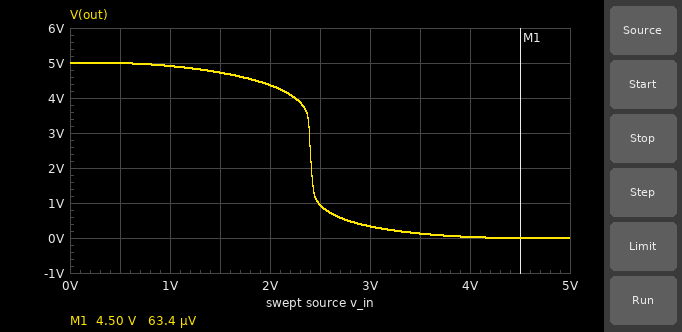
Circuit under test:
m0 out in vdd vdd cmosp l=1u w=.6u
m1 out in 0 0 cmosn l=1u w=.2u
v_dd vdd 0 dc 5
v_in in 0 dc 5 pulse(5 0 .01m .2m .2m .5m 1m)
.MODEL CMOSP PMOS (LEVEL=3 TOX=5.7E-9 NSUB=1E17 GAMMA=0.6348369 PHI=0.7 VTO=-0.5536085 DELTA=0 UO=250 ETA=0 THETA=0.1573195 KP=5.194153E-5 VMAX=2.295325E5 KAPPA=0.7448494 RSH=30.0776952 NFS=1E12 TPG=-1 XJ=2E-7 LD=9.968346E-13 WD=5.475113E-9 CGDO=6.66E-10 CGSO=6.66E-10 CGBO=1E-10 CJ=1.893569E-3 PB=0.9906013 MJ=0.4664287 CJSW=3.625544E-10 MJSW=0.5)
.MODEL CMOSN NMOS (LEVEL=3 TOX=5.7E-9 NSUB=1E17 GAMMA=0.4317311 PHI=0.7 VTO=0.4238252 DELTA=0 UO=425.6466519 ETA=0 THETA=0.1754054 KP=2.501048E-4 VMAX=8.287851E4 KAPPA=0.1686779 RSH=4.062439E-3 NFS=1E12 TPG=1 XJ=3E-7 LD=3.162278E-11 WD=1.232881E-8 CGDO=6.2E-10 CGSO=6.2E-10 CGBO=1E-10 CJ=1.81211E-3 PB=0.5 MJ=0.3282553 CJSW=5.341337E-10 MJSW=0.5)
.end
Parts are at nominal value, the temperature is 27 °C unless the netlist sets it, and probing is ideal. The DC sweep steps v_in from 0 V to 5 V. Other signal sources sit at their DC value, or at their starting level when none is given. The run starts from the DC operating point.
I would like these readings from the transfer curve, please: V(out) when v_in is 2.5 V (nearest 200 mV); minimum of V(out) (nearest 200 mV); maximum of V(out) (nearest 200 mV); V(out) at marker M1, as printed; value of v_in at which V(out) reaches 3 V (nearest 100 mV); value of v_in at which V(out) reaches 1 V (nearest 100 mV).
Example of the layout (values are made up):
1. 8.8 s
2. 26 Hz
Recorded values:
1. 1.0 V
2. 0 V
3. 5.0 V
4. 63.4 µV
5. 2.4 V
6. 2.5 V
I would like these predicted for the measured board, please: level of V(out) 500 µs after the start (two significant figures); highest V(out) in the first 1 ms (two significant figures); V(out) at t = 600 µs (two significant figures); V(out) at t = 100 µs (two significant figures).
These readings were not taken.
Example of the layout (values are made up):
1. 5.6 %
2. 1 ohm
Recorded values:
1. 5.0 V
2. 5.0 V
3. 5.0 V
4. 530 mV
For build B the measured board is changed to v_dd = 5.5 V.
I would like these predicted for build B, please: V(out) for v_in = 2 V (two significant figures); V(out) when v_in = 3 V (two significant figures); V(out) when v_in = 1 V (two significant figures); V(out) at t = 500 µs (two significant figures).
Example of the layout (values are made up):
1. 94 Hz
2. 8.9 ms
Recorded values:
1. 5.0 V
2. 650 mV
3. 5.4 V
4. 5.5 V
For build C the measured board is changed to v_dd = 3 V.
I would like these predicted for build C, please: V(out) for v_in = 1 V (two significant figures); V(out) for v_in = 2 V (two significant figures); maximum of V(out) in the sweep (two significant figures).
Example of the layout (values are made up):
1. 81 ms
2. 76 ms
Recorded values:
1. 2.8 V
2. 53 mV
3. 3.0 V
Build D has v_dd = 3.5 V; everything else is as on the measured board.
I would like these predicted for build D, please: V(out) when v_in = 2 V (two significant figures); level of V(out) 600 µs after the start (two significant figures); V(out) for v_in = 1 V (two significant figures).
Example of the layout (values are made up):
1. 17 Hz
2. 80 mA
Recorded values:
1. 220 mV
2. 3.5 V
3. 3.4 V
